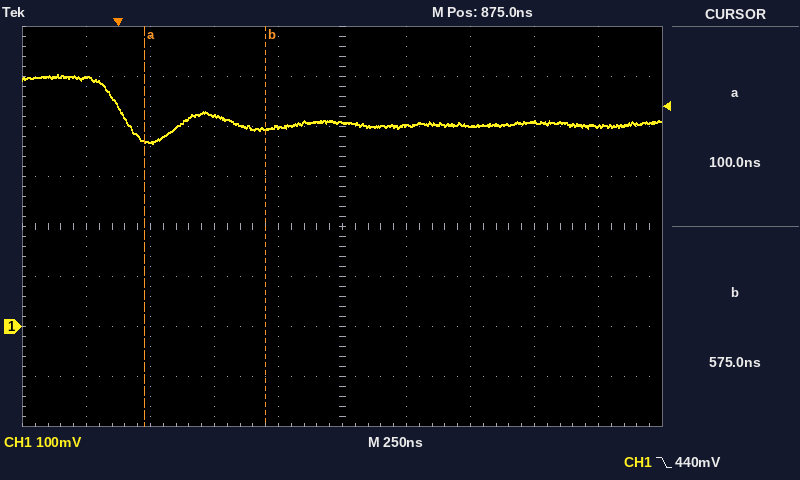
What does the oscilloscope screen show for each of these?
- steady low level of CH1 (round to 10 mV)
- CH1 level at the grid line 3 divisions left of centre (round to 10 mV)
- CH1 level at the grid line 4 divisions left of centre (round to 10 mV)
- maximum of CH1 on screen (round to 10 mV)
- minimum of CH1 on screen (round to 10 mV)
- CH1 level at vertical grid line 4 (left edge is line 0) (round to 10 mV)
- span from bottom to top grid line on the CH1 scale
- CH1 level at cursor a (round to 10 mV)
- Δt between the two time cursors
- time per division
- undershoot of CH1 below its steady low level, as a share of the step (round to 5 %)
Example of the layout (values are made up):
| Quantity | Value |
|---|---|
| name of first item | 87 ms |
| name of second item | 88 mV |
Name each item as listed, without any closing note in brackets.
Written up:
| Quantity | Value |
|---|---|
| steady low level of CH1 | 400 mV |
| CH1 level at the grid line 3 divisions left of centre | 370 mV |
| CH1 level at the grid line 4 divisions left of centre | 500 mV |
| maximum of CH1 on screen | 500 mV |
| minimum of CH1 on screen | 370 mV |
| CH1 level at vertical grid line 4 (left edge is line 0) | 400 mV |
| span from bottom to top grid line on the CH1 scale | 800 mV |
| CH1 level at cursor a | 370 mV |
| Δt between the two time cursors | 475 ns |
| time per division | 250 ns |
| undershoot of CH1 below its steady low level, as a share of the step | 40 % |
